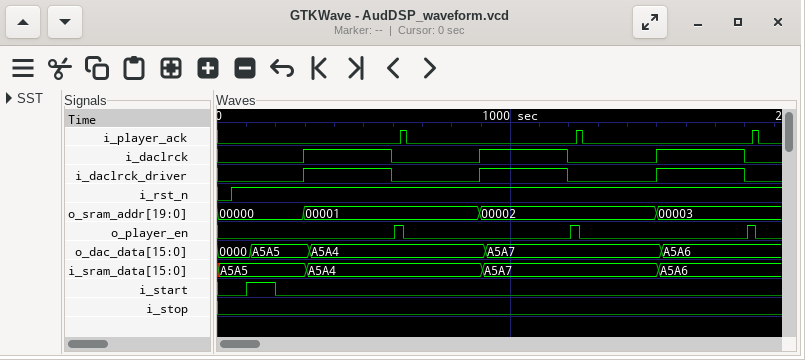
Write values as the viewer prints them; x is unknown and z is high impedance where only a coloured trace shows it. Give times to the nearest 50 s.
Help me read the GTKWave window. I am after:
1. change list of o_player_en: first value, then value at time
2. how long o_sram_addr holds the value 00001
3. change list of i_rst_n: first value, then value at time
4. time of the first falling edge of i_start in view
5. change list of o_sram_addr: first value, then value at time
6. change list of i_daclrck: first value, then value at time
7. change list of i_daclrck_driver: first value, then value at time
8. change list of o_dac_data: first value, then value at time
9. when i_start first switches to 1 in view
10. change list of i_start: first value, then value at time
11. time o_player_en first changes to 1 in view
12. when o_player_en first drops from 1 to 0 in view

0, 1 at 600 s, 0 at 650 s, 1 at 1200 s, 0 at 1250 s, 1 at 1800 s, 0 at 1850 s
600 s
0, 1 at 50 s
200 s
00000, 00001 at 300 s, 00002 at 900 s, 00003 at 1500 s
0, 1 at 300 s, 0 at 600 s, 1 at 900 s, 0 at 1200 s, 1 at 1500 s, 0 at 1800 s
0, 1 at 300 s, 0 at 600 s, 1 at 900 s, 0 at 1200 s, 1 at 1500 s, 0 at 1800 s
0000, A5A5 at 100 s, A5A4 at 300 s, A5A7 at 900 s, A5A6 at 1500 s
100 s
0, 1 at 100 s, 0 at 200 s
600 s
650 s
